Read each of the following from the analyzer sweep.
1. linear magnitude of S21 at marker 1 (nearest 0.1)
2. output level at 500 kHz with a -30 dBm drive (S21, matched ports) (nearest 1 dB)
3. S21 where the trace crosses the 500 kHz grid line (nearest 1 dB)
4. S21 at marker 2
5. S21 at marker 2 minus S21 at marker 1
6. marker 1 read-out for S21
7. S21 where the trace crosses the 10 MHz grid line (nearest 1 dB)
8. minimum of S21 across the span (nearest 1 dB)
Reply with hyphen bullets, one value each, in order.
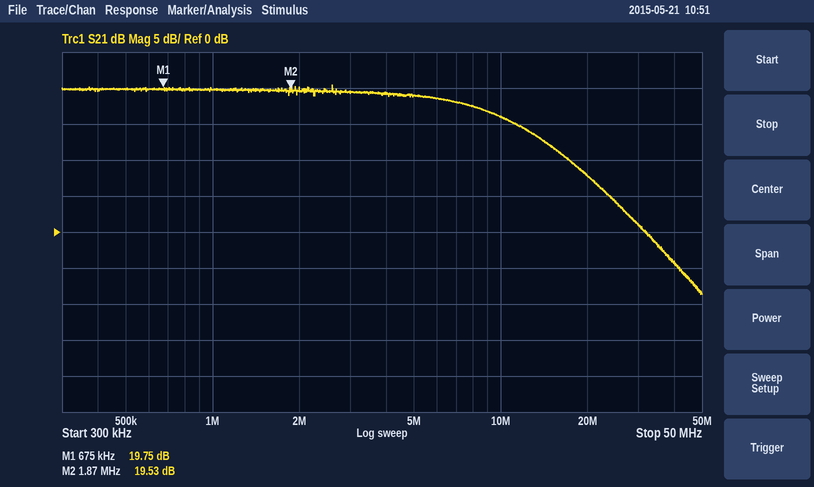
- 9.7
- -10 dBm
- 20 dB
- 19.53 dB
- -0.22 dB
- 19.75 dB
- 16 dB
- -9 dB
